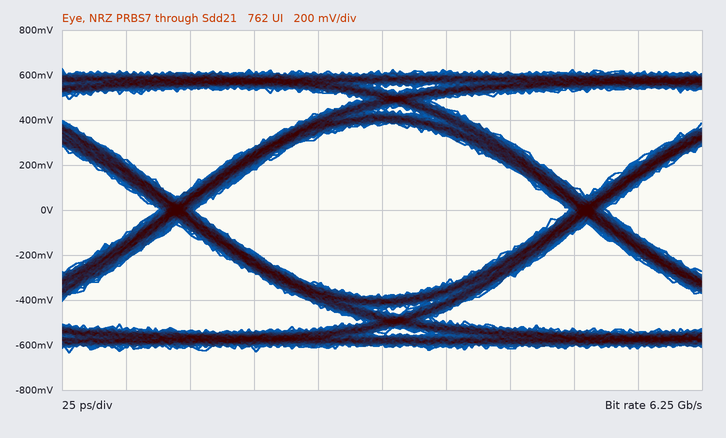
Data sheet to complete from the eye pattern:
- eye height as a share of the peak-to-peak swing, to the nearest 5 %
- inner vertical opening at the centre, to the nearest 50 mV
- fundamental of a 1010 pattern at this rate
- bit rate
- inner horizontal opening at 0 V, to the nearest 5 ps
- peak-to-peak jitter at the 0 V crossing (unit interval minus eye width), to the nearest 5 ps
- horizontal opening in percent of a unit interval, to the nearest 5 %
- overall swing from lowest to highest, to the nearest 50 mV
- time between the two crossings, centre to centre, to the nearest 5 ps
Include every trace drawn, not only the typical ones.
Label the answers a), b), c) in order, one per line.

a) 60 %
b) 750 mV
c) 3.125 GHz
d) 6.25 Gb/s
e) 145 ps
f) 15 ps
g) 90 %
h) 1.25 V
i) 160 ps
